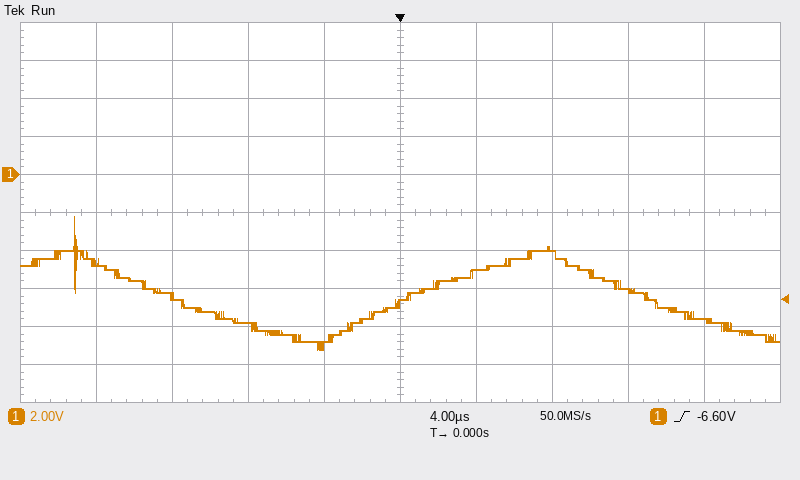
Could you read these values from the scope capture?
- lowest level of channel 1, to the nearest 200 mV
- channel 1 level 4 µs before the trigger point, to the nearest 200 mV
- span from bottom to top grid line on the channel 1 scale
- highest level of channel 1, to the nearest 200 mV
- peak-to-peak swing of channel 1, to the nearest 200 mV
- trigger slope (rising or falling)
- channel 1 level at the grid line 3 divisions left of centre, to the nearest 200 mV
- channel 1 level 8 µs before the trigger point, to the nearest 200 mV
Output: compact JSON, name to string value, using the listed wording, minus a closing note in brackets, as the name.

{"lowest level of channel 1, to the nearest 200 mV": "-9.2 V", "channel 1 level 4 µs before the trigger point, to the nearest 200 mV": "-9.0 V", "span from bottom to top grid line on the channel 1 scale": "20 V", "highest level of channel 1, to the nearest 200 mV": "-2.2 V", "peak-to-peak swing of channel 1, to the nearest 200 mV": "7.0 V", "trigger slope": "rising", "channel 1 level at the grid line 3 divisions left of centre, to the nearest 200 mV": "-6.4 V", "channel 1 level 8 µs before the trigger point, to the nearest 200 mV": "-8.0 V"}
